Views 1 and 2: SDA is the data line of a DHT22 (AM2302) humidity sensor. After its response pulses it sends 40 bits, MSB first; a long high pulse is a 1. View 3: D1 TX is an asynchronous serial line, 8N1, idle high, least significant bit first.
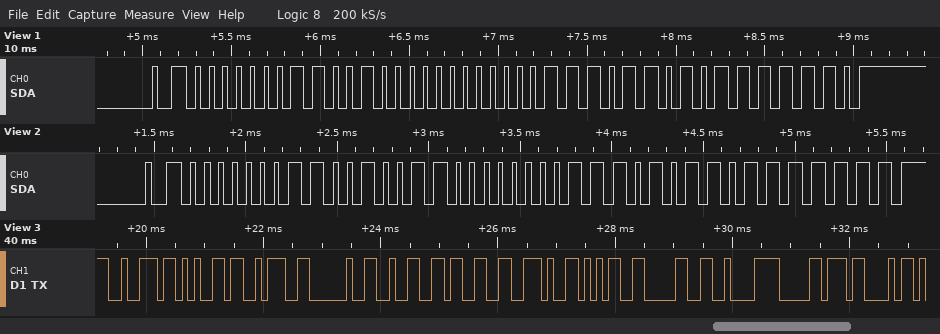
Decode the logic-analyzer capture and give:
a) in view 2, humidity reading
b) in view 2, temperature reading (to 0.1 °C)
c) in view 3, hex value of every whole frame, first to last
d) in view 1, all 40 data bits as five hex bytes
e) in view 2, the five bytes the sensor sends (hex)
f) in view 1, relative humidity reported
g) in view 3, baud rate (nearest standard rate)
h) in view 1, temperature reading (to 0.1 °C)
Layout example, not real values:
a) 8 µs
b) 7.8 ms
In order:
a) 40.3 %
b) 23.5 °C
c) 72 65 3A 20 32 33 2E 35 30 C2 B0 43
d) 01 90 00 ED 7E
e) 01 93 00 EB 7F
f) 40.0 %
g) 9600 baud
h) 23.7 °C
